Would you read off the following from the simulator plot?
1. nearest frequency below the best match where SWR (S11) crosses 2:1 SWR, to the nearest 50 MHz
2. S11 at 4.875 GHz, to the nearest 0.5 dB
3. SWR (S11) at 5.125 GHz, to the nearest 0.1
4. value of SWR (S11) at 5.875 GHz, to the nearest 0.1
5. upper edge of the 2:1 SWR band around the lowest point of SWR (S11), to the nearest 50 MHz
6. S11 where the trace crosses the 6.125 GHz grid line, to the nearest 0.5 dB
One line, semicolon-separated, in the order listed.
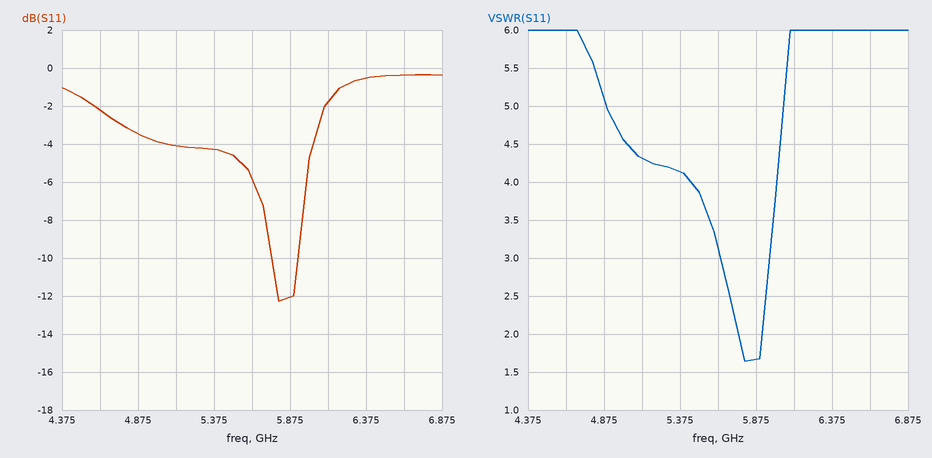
5.75 GHz; -3.5 dB; 4.3; 1.7; 5.90 GHz; -2.0 dB
